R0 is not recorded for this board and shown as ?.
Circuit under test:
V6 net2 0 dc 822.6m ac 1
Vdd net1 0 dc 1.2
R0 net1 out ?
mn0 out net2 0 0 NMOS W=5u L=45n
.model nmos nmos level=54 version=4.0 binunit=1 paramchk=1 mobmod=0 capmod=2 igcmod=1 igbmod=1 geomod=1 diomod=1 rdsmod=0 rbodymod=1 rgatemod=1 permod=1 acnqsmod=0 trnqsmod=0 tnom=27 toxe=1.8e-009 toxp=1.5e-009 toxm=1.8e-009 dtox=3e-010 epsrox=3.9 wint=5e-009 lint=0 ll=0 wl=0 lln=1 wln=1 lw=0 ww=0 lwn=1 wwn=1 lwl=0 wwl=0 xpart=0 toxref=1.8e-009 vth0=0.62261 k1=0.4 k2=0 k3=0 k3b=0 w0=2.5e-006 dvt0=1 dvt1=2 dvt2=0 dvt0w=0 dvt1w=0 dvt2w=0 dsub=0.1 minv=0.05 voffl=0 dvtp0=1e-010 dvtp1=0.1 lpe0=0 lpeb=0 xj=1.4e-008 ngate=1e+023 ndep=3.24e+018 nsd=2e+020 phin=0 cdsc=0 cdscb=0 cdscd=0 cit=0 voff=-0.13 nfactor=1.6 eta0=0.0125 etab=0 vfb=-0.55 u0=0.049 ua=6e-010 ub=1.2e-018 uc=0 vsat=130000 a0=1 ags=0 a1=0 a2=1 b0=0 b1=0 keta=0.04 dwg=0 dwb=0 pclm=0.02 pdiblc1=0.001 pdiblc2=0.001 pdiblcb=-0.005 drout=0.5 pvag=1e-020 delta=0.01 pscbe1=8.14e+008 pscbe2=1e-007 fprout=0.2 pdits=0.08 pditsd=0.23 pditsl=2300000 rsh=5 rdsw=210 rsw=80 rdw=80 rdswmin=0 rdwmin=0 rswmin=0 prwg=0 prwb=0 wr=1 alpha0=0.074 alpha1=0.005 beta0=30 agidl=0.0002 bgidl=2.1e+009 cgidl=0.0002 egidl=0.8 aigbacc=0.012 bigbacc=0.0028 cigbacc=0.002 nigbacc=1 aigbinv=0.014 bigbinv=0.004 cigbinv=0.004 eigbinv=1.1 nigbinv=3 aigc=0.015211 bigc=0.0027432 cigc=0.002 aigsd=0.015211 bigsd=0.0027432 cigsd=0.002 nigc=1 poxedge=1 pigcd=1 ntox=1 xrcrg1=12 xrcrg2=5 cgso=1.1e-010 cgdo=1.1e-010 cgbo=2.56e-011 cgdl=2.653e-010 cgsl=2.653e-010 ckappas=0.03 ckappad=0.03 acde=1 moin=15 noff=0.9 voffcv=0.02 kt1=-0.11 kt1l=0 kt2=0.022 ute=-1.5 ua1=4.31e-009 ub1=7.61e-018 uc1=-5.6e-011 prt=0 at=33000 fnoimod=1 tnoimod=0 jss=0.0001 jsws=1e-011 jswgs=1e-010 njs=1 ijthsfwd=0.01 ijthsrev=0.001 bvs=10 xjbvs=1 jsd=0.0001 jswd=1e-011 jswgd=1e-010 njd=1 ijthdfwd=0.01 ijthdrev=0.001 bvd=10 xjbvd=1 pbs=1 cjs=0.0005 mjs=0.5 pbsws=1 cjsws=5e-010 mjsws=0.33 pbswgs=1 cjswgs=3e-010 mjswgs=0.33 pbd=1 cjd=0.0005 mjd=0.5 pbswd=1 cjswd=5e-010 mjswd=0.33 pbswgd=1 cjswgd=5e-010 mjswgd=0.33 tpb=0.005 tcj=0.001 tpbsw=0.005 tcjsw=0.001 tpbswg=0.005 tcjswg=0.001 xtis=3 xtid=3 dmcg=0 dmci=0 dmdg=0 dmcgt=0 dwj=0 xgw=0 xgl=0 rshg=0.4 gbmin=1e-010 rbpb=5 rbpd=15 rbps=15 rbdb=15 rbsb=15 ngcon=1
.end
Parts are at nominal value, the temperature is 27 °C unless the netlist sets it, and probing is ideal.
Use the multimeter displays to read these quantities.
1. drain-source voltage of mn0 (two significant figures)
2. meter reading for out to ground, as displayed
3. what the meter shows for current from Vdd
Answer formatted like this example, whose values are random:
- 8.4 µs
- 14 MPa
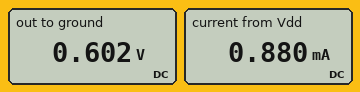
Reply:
- 600 mV
- 0.602 V
- 0.880 mA
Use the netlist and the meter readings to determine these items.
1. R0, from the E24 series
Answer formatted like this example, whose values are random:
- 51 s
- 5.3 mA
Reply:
- 680 Ω
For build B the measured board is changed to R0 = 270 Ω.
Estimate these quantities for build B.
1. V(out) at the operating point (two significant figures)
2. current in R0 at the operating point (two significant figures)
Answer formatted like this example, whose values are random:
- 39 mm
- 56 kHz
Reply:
- 930 mV
- 1.0 mA
